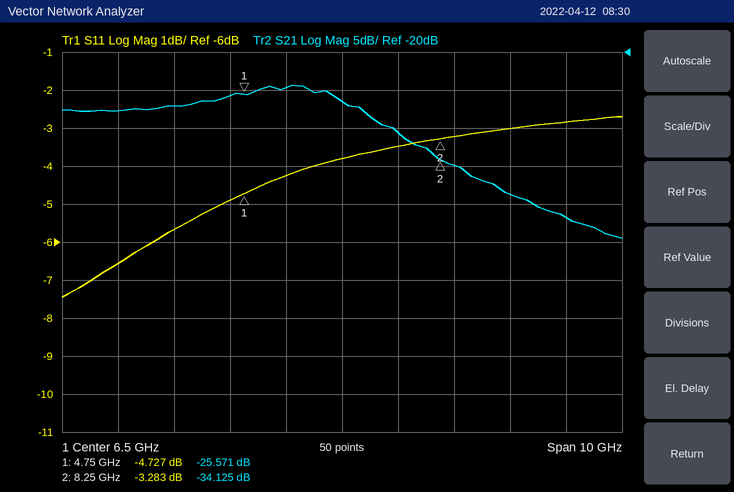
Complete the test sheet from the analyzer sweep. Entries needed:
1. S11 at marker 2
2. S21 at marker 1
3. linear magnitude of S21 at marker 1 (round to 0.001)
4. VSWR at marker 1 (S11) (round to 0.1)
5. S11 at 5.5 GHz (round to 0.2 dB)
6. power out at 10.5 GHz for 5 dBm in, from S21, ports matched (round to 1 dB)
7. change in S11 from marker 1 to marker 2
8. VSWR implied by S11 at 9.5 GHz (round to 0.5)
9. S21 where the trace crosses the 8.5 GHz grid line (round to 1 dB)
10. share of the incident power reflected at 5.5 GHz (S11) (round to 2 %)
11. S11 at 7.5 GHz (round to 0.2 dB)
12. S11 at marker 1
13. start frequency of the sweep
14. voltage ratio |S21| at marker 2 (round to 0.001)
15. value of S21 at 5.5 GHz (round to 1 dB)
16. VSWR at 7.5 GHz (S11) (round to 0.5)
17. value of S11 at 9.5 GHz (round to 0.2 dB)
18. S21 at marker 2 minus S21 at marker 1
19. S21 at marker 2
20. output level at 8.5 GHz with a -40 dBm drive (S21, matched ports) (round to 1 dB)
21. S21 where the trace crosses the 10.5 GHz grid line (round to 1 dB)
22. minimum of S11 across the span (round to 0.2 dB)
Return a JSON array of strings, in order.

["-3.283 dB", "-25.571 dB", "0.053", "3.8", "-4.2 dB", "-37 dBm", "1.444 dB", "6.0", "-35 dB", "38 %", "-3.4 dB", "-4.727 dB", "1.5 GHz", "0.020", "-25 dB", "5.0", "-3.0 dB", "-8.554 dB", "-34.125 dB", "-75 dBm", "-42 dB", "-7.4 dB"]
